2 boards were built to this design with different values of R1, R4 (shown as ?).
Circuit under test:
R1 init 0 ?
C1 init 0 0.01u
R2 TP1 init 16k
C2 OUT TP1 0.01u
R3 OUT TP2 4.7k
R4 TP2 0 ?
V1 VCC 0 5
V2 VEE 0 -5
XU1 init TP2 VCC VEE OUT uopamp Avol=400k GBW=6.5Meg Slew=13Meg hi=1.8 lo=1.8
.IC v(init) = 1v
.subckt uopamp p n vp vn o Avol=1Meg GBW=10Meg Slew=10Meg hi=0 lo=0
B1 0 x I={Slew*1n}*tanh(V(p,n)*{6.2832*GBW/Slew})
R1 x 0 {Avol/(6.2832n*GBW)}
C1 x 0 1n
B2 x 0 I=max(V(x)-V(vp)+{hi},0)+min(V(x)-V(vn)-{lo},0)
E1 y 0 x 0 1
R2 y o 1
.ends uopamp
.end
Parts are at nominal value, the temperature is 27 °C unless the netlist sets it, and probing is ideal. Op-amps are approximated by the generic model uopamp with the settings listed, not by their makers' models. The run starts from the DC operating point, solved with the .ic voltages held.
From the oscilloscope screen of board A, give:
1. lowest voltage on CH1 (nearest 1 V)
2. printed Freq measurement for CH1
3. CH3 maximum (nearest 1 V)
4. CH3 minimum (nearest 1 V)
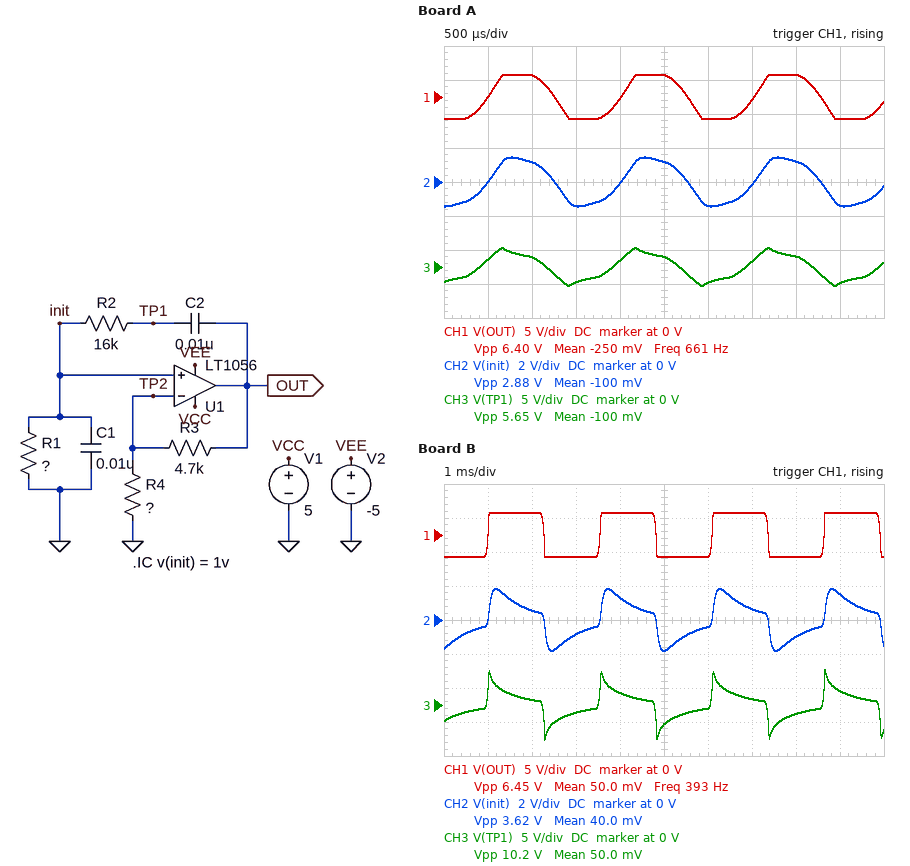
-3 V
661 Hz
3 V
-3 V
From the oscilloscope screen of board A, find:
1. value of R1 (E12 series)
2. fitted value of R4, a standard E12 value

33 kΩ
2.7 kΩ
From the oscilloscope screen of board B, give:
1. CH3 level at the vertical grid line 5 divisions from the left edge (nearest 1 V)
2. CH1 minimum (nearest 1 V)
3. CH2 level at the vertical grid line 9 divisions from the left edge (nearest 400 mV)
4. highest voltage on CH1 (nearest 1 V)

-3 V
-3 V
1.6 V
3 V
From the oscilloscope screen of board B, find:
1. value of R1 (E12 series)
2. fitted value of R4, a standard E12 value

27 kΩ
680 Ω
